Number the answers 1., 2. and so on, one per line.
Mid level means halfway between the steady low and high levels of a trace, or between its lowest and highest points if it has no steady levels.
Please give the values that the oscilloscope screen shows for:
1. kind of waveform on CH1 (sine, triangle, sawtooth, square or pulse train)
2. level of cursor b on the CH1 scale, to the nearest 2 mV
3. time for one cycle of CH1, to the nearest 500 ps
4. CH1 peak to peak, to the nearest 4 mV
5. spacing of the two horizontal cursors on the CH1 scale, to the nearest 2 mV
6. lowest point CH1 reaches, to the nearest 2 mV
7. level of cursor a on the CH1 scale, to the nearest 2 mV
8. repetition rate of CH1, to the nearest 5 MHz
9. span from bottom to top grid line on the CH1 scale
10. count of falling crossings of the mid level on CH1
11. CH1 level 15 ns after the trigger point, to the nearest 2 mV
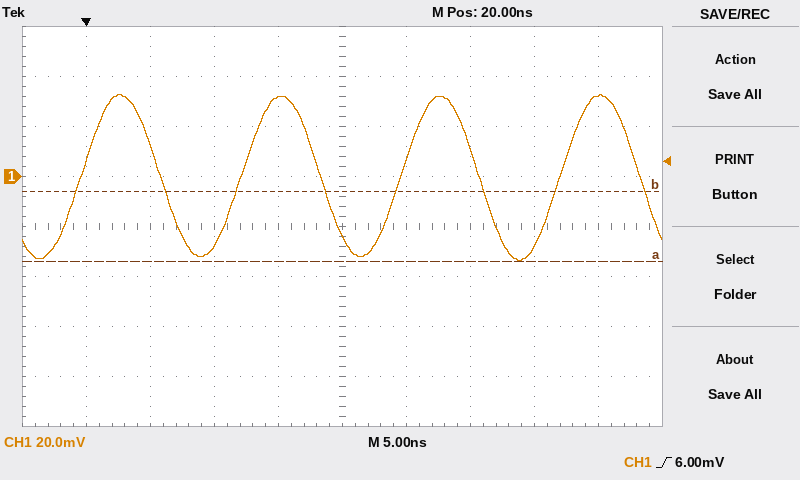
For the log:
1. sine
2. -6 mV
3. 12.5 ns
4. 68 mV
5. 28 mV
6. -34 mV
7. -34 mV
8. 80 MHz
9. 160 mV
10. 4
11. 32 mV
